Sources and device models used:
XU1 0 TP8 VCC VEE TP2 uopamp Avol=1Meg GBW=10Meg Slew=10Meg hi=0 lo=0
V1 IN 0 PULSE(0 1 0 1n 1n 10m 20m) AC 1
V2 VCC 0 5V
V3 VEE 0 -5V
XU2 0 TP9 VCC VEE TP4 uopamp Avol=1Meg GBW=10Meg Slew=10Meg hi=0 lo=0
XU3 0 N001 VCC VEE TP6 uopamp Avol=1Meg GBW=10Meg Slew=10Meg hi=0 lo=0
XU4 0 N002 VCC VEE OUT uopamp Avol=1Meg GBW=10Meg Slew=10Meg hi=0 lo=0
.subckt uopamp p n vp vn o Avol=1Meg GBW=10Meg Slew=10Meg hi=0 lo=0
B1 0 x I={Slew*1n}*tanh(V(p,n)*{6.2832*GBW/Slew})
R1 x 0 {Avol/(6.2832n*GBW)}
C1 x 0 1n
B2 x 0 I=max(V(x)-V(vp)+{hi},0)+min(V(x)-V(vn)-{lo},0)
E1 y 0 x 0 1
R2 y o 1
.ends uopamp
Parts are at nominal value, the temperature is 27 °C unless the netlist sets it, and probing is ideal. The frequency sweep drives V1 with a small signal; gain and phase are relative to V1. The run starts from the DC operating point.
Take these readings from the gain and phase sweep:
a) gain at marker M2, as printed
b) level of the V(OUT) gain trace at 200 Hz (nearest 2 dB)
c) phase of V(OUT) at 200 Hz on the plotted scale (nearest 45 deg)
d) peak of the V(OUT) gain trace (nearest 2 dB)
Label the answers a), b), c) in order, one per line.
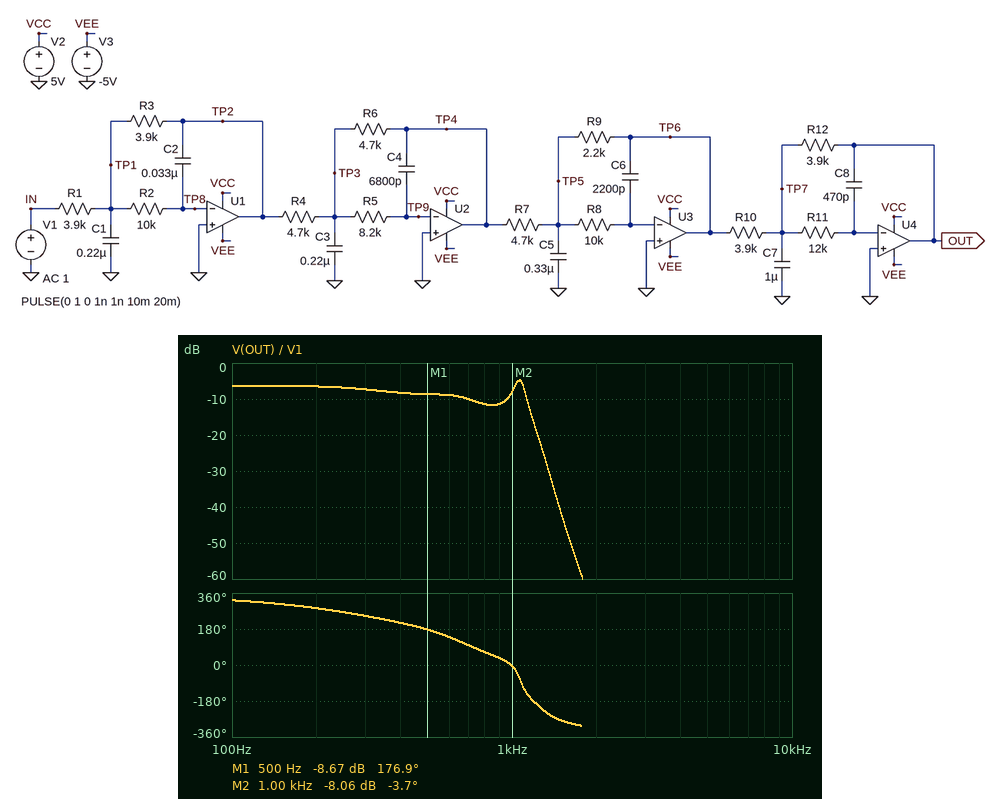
a) -8.06 dB
b) -6 dB
c) 270 deg
d) -4 dB
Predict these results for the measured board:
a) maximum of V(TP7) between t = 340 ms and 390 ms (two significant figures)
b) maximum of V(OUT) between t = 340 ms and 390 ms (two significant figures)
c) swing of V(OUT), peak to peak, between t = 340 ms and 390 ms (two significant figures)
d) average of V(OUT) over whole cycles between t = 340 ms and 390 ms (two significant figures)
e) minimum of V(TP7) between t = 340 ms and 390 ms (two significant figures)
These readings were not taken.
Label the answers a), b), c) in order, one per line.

a) 4.9 mV
b) 510 mV
c) 550 mV
d) 230 mV
e) -4.9 mV
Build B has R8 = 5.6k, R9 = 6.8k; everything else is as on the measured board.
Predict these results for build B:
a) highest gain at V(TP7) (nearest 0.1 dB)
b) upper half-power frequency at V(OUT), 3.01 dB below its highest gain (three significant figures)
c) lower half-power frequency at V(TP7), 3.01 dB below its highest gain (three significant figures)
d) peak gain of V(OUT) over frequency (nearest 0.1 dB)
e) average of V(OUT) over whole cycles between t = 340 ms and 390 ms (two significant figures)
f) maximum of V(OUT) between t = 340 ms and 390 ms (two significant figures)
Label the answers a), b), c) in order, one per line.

a) -23.0 dB
b) 1.09 kHz
c) 896 Hz
d) 5.6 dB
e) 720 mV
f) 1.7 V
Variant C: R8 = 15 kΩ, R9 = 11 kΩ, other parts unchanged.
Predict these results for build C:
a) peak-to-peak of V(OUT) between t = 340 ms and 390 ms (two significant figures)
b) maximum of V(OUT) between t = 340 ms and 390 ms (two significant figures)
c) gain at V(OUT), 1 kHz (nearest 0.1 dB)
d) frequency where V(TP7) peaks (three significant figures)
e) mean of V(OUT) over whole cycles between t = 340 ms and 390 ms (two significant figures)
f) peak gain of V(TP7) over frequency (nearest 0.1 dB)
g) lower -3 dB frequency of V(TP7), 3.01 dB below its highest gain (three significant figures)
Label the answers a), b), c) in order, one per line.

a) 4.2 V
b) 3.3 V
c) -12.9 dB
d) 452 Hz
e) 1.2 V
f) -23.3 dB
g) 362 Hz
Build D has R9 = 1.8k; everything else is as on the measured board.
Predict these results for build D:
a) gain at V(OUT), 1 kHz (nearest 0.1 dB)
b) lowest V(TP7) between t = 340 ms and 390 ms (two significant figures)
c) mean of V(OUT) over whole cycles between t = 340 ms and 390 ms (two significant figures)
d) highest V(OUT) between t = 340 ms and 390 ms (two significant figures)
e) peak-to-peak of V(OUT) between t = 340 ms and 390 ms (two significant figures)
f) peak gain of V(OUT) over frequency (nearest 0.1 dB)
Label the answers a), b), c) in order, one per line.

a) -11.5 dB
b) -3.9 mV
c) 190 mV
d) 410 mV
e) 440 mV
f) -8.2 dB
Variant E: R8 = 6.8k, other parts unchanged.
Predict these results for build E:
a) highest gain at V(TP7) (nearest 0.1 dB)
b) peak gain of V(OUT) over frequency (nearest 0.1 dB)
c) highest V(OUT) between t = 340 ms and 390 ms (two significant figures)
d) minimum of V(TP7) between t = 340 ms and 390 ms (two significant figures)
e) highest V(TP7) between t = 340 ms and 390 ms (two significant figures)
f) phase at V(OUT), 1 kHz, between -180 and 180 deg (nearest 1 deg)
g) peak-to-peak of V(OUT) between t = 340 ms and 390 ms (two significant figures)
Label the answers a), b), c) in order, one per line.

a) -36.2 dB
b) -6.4 dB
c) 500 mV
d) -4.6 mV
e) 4.6 mV
f) 12 deg
g) 530 mV
